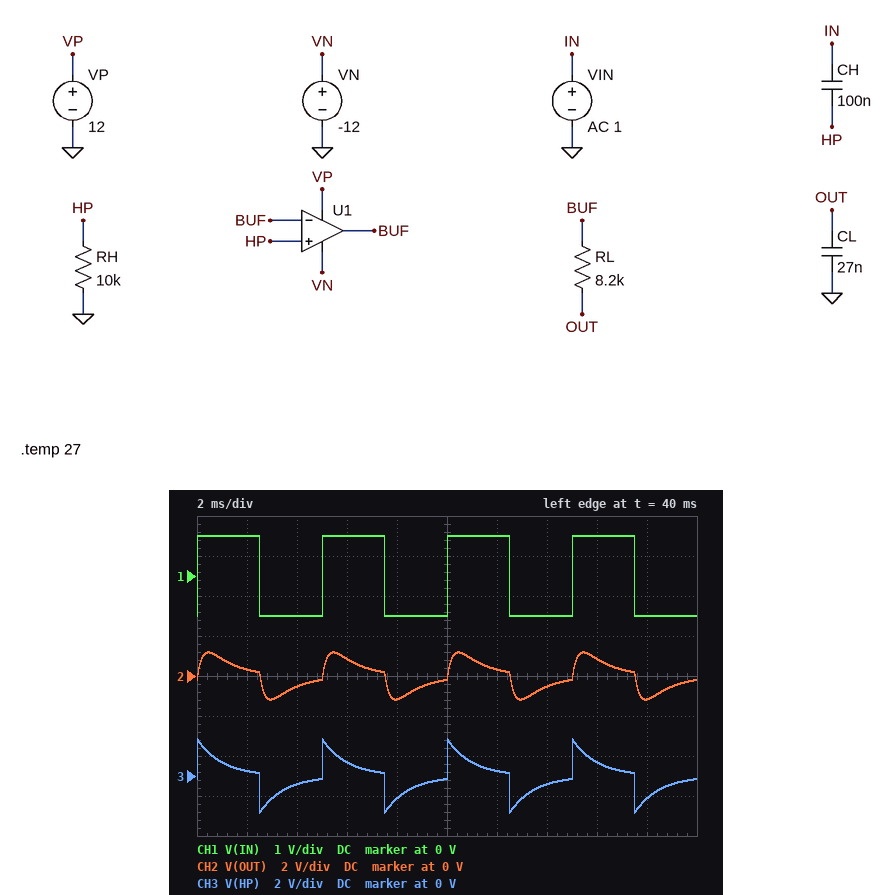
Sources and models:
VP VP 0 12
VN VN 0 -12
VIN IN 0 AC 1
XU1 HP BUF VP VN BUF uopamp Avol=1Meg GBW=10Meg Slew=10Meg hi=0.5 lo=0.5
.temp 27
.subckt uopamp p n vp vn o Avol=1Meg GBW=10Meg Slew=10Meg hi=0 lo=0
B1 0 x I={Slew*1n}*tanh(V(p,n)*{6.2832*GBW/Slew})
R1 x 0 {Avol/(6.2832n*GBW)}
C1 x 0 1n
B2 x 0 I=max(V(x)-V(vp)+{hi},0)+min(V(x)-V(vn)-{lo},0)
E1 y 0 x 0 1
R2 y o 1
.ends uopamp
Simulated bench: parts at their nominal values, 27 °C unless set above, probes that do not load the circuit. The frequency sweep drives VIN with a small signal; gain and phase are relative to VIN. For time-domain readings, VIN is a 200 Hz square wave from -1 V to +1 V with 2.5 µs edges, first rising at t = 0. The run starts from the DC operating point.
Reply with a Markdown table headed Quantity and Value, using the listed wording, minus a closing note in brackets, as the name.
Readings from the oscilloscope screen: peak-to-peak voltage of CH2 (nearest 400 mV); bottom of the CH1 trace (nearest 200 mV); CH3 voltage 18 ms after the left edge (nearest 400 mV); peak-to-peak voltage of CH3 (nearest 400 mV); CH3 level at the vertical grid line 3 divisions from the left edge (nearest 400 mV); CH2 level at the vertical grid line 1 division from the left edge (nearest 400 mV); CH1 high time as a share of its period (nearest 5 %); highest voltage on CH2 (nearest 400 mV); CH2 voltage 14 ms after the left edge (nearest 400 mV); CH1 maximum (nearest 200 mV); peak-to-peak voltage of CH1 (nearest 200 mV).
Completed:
| Quantity | Value |
|---|---|
| peak-to-peak voltage of CH2 | 2.4 V |
| bottom of the CH1 trace | -1.0 V |
| CH3 voltage 18 ms after the left edge | -1.2 V |
| peak-to-peak voltage of CH3 | 3.6 V |
| CH3 level at the vertical grid line 3 divisions from the left edge | 800 mV |
| CH2 level at the vertical grid line 1 division from the left edge | 400 mV |
| CH1 high time as a share of its period | 50 % |
| highest voltage on CH2 | 1.2 V |
| CH2 voltage 14 ms after the left edge | -400 mV |
| CH1 maximum | 1.0 V |
| peak-to-peak voltage of CH1 | 2.0 V |
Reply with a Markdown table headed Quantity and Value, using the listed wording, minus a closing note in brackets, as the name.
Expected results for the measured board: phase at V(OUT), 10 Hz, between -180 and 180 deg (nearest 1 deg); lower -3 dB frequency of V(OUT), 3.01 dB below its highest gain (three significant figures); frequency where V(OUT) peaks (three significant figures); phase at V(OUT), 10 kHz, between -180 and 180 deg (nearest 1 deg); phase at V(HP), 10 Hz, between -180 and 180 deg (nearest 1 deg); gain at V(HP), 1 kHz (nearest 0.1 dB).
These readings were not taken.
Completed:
| Quantity | Value |
|---|---|
| phase at V(OUT), 10 Hz, between -180 and 180 deg | 86 deg |
| lower -3 dB frequency of V(OUT), 3.01 dB below its highest gain | 115 Hz |
| frequency where V(OUT) peaks | 338 Hz |
| phase at V(OUT), 10 kHz, between -180 and 180 deg | -85 deg |
| phase at V(HP), 10 Hz, between -180 and 180 deg | 86 deg |
| gain at V(HP), 1 kHz | -0.1 dB |
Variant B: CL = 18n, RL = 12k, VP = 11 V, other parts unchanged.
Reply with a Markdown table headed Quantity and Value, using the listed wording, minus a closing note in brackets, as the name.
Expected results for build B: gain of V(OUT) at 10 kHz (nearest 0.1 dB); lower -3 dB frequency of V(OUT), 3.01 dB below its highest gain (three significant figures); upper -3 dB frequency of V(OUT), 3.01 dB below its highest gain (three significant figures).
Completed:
| Quantity | Value |
|---|---|
| gain of V(OUT) at 10 kHz | -22.7 dB |
| lower -3 dB frequency of V(OUT), 3.01 dB below its highest gain | 116 Hz |
| upper -3 dB frequency of V(OUT), 3.01 dB below its highest gain | 1.01 kHz |
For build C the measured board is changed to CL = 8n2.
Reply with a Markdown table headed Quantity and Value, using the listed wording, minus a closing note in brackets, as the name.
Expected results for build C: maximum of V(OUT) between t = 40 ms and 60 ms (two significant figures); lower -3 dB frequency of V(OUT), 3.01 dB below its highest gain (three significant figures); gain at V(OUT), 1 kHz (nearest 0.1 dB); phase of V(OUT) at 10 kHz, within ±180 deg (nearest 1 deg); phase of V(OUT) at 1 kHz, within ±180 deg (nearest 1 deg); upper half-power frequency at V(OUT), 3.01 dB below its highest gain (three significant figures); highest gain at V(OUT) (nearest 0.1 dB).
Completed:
| Quantity | Value |
|---|---|
| maximum of V(OUT) between t = 40 ms and 60 ms | 1.5 V |
| lower -3 dB frequency of V(OUT), 3.01 dB below its highest gain | 141 Hz |
| gain at V(OUT), 1 kHz | -0.8 dB |
| phase of V(OUT) at 10 kHz, within ±180 deg | -76 deg |
| phase of V(OUT) at 1 kHz, within ±180 deg | -14 deg |
| upper half-power frequency at V(OUT), 3.01 dB below its highest gain | 2.67 kHz |
| highest gain at V(OUT) | -0.6 dB |
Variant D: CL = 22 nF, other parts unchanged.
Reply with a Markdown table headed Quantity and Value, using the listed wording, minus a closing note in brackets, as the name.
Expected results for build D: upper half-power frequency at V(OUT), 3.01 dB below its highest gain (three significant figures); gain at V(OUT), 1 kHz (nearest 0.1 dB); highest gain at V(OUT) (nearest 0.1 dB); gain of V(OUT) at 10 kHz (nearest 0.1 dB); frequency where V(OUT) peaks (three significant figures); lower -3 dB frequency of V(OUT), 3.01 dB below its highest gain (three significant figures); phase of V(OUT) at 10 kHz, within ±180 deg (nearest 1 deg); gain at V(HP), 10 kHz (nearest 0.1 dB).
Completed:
| Quantity | Value |
|---|---|
| upper half-power frequency at V(OUT), 3.01 dB below its highest gain | 1.16 kHz |
| gain at V(OUT), 1 kHz | -3.7 dB |
| highest gain at V(OUT) | -1.4 dB |
| gain of V(OUT) at 10 kHz | -21.1 dB |
| frequency where V(OUT) peaks | 375 Hz |
| lower -3 dB frequency of V(OUT), 3.01 dB below its highest gain | 121 Hz |
| phase of V(OUT) at 10 kHz, within ±180 deg | -84 deg |
| gain at V(HP), 10 kHz | 0 dB |
